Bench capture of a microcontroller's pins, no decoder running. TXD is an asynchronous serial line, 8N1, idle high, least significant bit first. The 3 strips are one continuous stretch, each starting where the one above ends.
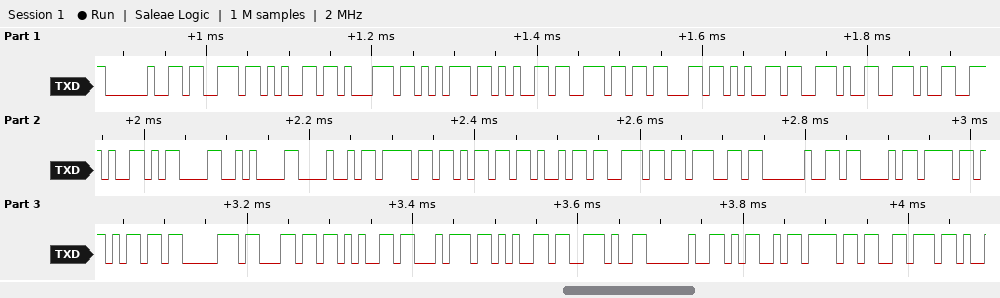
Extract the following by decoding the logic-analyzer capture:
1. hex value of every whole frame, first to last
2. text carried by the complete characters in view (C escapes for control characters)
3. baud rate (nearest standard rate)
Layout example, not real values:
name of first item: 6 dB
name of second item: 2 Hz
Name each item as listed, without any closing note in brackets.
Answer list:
hex value of every whole frame, first to last: 20 73 65 71 75 65 6E 63 65 2E 2E 2E 0D 0A 48 6F 6D 69 6E 67 20 43 6F 6D 70 6C 65 74 65 2E 20 4D 6F 76
text carried by the complete characters in view: " sequence...\r\nHoming Complete. Mov"
baud rate: 115200 baud
